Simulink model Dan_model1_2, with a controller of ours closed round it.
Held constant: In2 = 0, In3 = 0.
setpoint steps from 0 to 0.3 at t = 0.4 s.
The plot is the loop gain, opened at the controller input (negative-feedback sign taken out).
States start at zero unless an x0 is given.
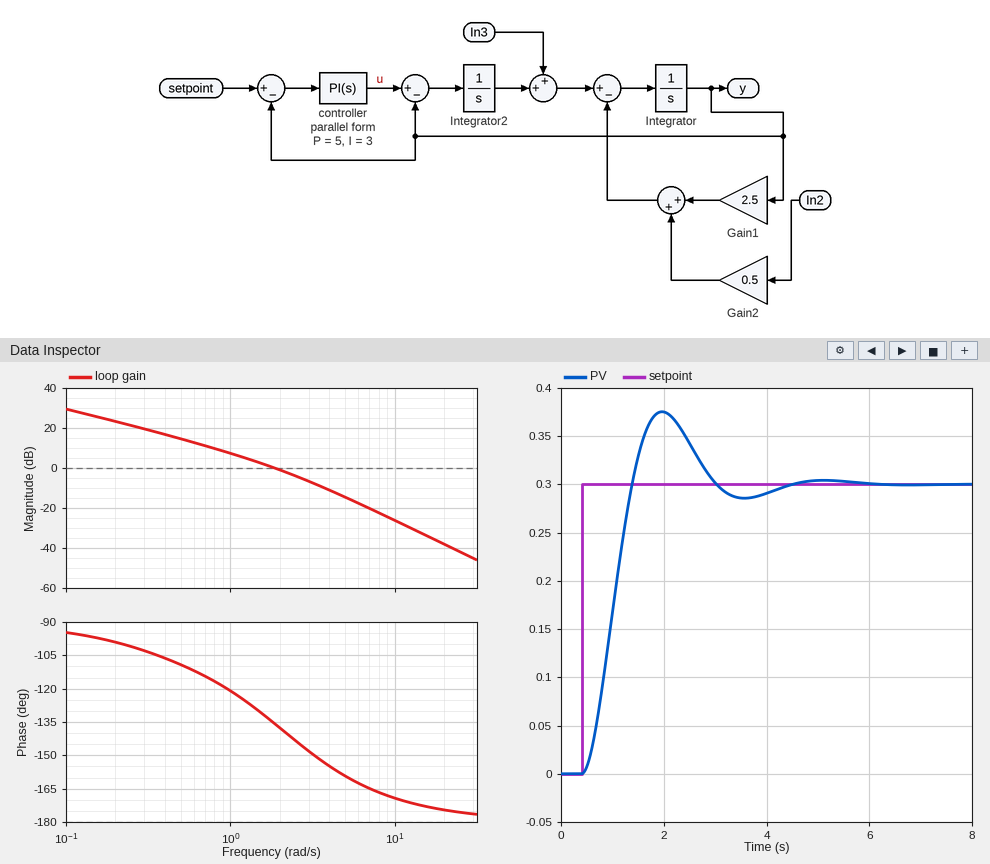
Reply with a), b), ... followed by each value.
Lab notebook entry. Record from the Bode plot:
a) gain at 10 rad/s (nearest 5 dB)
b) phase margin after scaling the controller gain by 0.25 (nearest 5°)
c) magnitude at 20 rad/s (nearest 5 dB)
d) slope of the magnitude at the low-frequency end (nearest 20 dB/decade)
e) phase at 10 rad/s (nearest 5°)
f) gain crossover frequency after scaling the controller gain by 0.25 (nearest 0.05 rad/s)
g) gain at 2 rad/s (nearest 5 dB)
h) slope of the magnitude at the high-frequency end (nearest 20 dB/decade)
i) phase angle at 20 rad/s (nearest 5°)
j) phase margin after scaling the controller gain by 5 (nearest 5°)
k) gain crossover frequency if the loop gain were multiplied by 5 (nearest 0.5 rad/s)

a) -25 dB
b) 65°
c) -40 dB
d) -20 dB/decade
e) -170°
f) 0.65 rad/s
g) 0 dB
h) -40 dB/decade
i) -175°
j) 20°
k) 5.0 rad/s
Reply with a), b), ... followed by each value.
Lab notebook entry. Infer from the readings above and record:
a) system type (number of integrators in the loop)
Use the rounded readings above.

a) 1
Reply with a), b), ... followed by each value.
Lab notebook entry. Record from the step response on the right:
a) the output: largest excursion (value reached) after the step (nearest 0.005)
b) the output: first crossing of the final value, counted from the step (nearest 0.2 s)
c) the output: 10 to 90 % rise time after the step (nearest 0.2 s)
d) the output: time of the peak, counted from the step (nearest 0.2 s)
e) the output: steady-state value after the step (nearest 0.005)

a) 0.375
b) 1.0 s
c) 0.6 s
d) 1.6 s
e) 0.300
